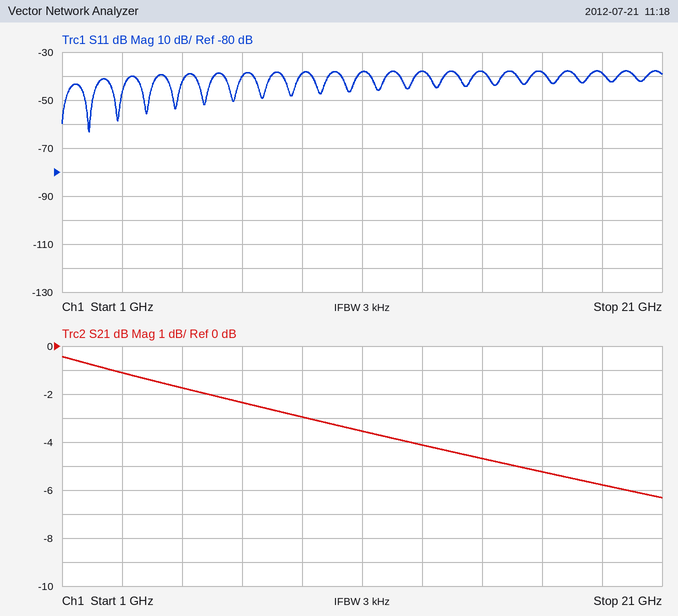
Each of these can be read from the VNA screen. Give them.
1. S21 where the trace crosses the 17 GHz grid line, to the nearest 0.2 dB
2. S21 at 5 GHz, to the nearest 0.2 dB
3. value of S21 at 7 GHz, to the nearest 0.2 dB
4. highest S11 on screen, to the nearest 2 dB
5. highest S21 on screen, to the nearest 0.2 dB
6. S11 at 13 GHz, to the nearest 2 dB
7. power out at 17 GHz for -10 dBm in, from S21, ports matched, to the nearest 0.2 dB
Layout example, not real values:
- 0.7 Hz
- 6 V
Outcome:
- -5.2 dB
- -1.8 dB
- -2.4 dB
- -38 dB
- -0.4 dB
- -38 dB
- -15.2 dBm
